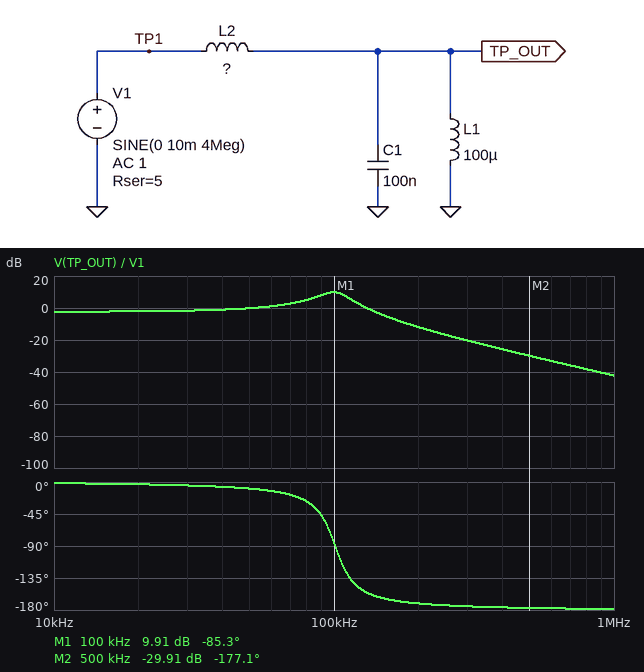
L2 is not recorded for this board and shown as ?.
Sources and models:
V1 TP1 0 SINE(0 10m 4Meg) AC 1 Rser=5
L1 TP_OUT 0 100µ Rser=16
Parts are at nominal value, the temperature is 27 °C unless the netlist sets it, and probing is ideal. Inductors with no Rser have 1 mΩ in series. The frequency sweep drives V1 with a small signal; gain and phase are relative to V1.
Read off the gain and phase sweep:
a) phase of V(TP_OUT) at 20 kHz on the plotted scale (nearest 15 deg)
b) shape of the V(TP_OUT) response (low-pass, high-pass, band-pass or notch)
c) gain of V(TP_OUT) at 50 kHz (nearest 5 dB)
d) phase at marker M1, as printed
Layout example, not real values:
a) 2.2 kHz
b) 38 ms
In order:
a) 0 deg
b) low-pass
c) 0 dB
d) -85.3 deg
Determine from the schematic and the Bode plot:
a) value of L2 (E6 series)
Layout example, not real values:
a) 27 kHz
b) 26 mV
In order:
a) 33 µH
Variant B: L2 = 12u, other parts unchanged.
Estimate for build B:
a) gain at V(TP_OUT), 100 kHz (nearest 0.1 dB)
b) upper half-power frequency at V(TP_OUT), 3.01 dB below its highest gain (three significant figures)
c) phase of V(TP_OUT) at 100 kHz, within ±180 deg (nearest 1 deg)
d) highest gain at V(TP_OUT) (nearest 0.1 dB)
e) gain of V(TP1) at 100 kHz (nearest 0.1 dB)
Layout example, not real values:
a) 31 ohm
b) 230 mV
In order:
a) 3.0 dB
b) 176 kHz
c) -22 deg
d) 7.1 dB
e) -0.9 dB
